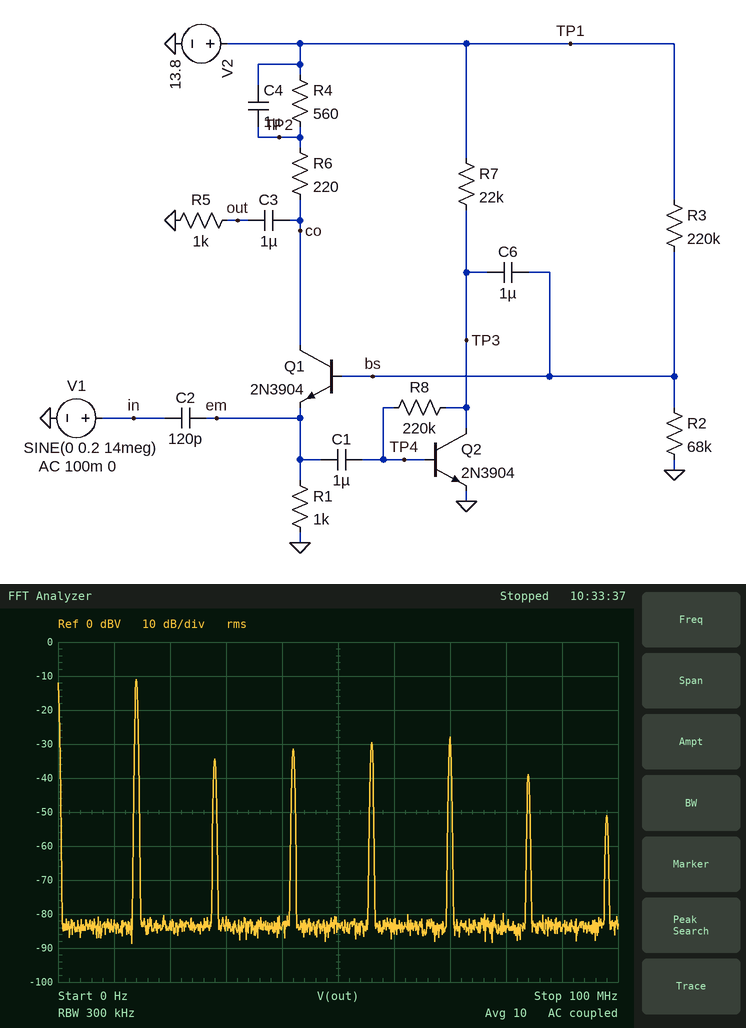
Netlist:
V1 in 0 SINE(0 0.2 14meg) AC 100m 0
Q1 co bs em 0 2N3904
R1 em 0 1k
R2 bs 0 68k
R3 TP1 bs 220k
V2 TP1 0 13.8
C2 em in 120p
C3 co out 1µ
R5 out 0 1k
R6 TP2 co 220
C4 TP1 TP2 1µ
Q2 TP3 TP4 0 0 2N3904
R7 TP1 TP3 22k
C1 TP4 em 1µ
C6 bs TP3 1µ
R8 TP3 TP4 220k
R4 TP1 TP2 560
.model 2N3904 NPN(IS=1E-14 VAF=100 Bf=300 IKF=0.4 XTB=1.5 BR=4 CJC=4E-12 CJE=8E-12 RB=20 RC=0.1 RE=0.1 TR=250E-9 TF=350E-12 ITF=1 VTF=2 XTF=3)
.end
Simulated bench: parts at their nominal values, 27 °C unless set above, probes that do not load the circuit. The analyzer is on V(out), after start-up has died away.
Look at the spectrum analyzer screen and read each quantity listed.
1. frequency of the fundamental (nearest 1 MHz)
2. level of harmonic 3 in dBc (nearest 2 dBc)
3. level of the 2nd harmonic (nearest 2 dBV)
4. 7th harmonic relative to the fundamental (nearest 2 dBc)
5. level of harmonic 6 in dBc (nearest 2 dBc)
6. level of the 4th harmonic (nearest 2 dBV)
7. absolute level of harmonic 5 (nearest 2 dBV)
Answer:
14 MHz
-20 dBc
-34 dBV
-40 dBc
-28 dBc
-30 dBV
-28 dBV
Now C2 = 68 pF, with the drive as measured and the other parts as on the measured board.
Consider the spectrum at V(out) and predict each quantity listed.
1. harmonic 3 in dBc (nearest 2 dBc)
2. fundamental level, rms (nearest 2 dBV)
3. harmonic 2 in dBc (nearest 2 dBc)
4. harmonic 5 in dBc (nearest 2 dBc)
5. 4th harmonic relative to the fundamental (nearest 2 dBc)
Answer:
-48 dBc
-16 dBV
-40 dBc
-58 dBc
-54 dBc
